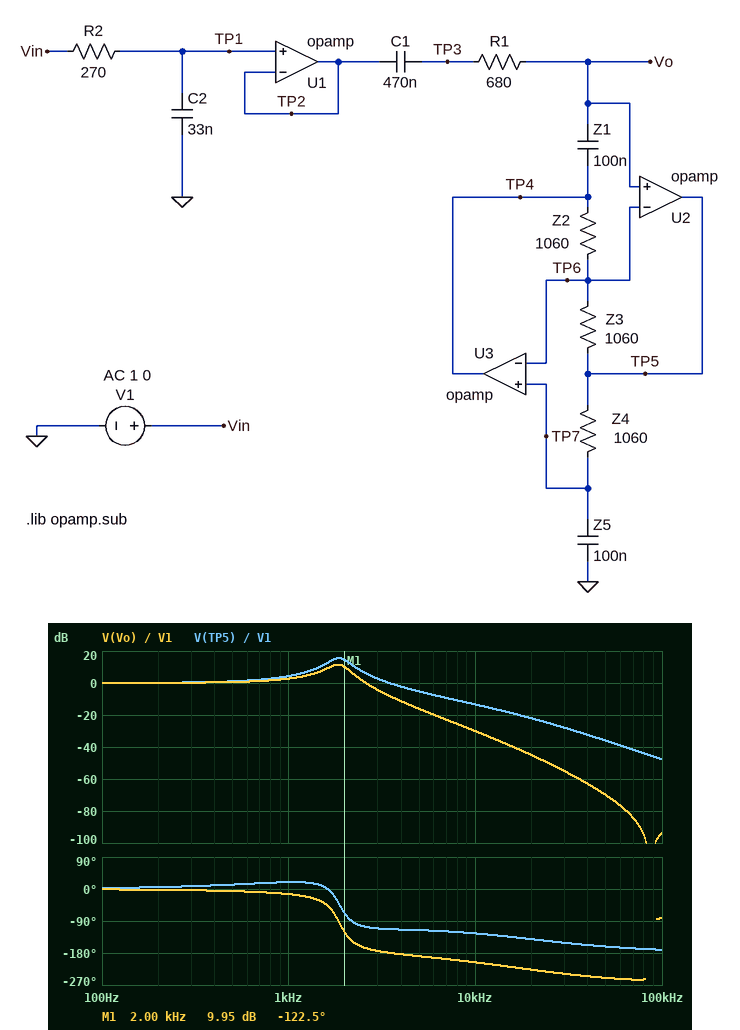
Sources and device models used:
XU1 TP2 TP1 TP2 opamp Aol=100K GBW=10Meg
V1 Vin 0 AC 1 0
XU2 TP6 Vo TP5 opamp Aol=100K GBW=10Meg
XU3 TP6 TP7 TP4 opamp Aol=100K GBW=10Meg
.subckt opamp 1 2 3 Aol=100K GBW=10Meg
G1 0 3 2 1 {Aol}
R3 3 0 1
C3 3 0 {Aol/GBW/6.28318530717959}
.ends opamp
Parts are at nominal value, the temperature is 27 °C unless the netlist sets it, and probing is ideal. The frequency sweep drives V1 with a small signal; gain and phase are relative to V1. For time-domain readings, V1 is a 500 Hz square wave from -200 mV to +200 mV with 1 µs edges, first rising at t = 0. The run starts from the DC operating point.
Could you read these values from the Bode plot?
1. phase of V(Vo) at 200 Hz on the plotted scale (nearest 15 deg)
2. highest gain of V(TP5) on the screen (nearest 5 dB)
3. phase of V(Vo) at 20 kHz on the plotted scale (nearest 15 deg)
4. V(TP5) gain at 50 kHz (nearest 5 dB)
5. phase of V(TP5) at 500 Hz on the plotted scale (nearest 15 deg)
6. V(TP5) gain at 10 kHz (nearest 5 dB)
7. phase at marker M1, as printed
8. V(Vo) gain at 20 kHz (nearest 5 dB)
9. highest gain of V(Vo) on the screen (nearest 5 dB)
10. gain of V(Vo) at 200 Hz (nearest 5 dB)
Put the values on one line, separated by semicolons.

0 deg; 15 dB; -225 deg; -35 dB; 15 deg; -15 dB; -122.5 deg; -45 dB; 10 dB; 0 dB
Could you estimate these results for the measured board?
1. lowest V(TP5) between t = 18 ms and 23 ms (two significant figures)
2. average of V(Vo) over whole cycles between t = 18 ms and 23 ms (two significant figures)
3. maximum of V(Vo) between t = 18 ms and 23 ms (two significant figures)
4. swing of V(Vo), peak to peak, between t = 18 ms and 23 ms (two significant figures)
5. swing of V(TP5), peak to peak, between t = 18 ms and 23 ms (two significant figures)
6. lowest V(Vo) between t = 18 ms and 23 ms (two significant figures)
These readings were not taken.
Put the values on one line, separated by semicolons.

-400 mV; 200 mV; 630 mV; 870 mV; 1.2 V; -230 mV
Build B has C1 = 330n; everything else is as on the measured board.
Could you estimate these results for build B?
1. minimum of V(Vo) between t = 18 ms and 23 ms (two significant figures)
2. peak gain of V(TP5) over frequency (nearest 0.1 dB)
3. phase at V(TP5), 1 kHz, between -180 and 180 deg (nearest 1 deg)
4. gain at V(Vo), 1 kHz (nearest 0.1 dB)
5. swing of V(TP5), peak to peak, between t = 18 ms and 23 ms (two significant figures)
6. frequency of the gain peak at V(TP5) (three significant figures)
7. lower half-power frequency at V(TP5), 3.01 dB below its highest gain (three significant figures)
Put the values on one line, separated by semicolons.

-210 mV; 12.5 dB; 15 deg; 2.6 dB; 1.1 V; 1.85 kHz; 1.50 kHz
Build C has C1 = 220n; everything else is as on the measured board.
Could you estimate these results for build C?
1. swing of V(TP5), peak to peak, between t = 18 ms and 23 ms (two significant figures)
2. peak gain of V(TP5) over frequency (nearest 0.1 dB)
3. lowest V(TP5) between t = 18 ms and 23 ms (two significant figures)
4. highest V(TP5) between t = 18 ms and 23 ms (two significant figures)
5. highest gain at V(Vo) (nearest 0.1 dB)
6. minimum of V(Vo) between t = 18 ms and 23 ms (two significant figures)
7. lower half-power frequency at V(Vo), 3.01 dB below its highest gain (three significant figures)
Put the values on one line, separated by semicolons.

990 mV; 9.0 dB; -290 mV; 690 mV; 5.2 dB; -160 mV; 1.01 kHz
